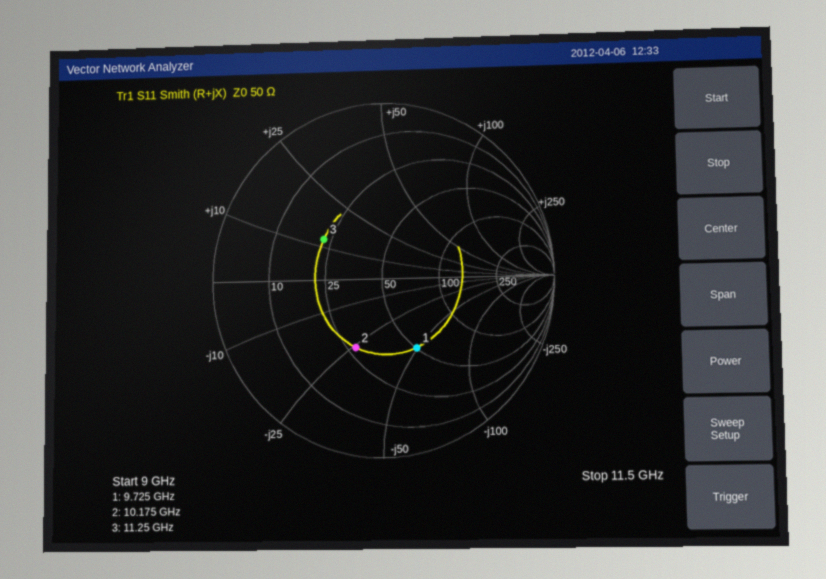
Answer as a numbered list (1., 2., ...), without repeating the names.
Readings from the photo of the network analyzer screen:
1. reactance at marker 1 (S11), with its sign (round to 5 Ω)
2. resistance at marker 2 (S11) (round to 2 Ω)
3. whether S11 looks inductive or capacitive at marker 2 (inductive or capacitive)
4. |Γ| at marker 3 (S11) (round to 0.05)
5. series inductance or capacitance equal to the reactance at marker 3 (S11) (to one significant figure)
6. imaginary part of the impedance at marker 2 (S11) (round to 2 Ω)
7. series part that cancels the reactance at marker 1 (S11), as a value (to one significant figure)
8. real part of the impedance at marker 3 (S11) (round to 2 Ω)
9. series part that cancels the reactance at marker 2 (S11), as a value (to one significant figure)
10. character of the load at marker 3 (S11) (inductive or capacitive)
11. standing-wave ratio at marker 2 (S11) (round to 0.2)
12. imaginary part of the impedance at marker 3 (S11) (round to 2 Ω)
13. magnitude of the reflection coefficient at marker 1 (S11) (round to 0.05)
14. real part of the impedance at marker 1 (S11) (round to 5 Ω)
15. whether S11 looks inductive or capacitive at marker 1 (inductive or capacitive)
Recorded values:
1. -50 Ω
2. 28 Ω
3. capacitive
4. 0.40
5. 200 pH
6. -26 Ω
7. 800 pH
8. 22 Ω
9. 400 pH
10. inductive
11. 2.4
12. +12 Ω
13. 0.45
14. 50 Ω
15. capacitive
